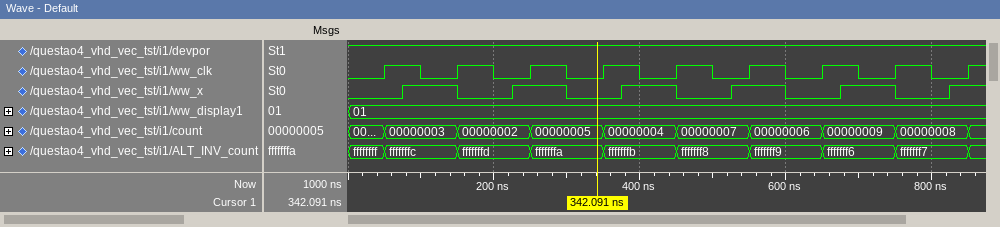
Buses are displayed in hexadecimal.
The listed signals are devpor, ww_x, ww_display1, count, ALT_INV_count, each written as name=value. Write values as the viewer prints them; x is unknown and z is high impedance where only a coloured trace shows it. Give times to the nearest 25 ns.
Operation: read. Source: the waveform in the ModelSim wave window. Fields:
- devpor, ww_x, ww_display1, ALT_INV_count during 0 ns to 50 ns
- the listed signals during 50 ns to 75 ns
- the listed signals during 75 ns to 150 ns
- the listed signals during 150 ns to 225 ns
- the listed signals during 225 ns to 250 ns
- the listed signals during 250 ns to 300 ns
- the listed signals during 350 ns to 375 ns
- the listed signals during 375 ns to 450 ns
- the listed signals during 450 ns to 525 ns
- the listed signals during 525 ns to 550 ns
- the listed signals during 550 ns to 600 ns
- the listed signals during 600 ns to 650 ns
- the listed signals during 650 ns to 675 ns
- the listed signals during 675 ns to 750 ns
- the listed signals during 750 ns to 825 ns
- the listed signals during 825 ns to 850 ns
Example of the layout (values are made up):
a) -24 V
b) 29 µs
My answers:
a) devpor=1, ww_x=0, ww_display1=01, ALT_INV_count=ffffffff
b) devpor=1, ww_x=0, ww_display1=01, count=00000003, ALT_INV_count=fffffffc
c) devpor=1, ww_x=1, ww_display1=01, count=00000003, ALT_INV_count=fffffffc
d) devpor=1, ww_x=0, ww_display1=01, count=00000002, ALT_INV_count=fffffffd
e) devpor=1, ww_x=1, ww_display1=01, count=00000002, ALT_INV_count=fffffffd
f) devpor=1, ww_x=1, ww_display1=01, count=00000005, ALT_INV_count=fffffffa
g) devpor=1, ww_x=0, ww_display1=01, count=00000004, ALT_INV_count=fffffffb
h) devpor=1, ww_x=1, ww_display1=01, count=00000004, ALT_INV_count=fffffffb
i) devpor=1, ww_x=0, ww_display1=01, count=00000007, ALT_INV_count=fffffff8
j) devpor=1, ww_x=1, ww_display1=01, count=00000007, ALT_INV_count=fffffff8
k) devpor=1, ww_x=1, ww_display1=01, count=00000006, ALT_INV_count=fffffff9
l) devpor=1, ww_x=0, ww_display1=01, count=00000006, ALT_INV_count=fffffff9
m) devpor=1, ww_x=0, ww_display1=01, count=00000009, ALT_INV_count=fffffff6
n) devpor=1, ww_x=1, ww_display1=01, count=00000009, ALT_INV_count=fffffff6
o) devpor=1, ww_x=0, ww_display1=01, count=00000008, ALT_INV_count=fffffff7
p) devpor=1, ww_x=1, ww_display1=01, count=00000008, ALT_INV_count=fffffff7
